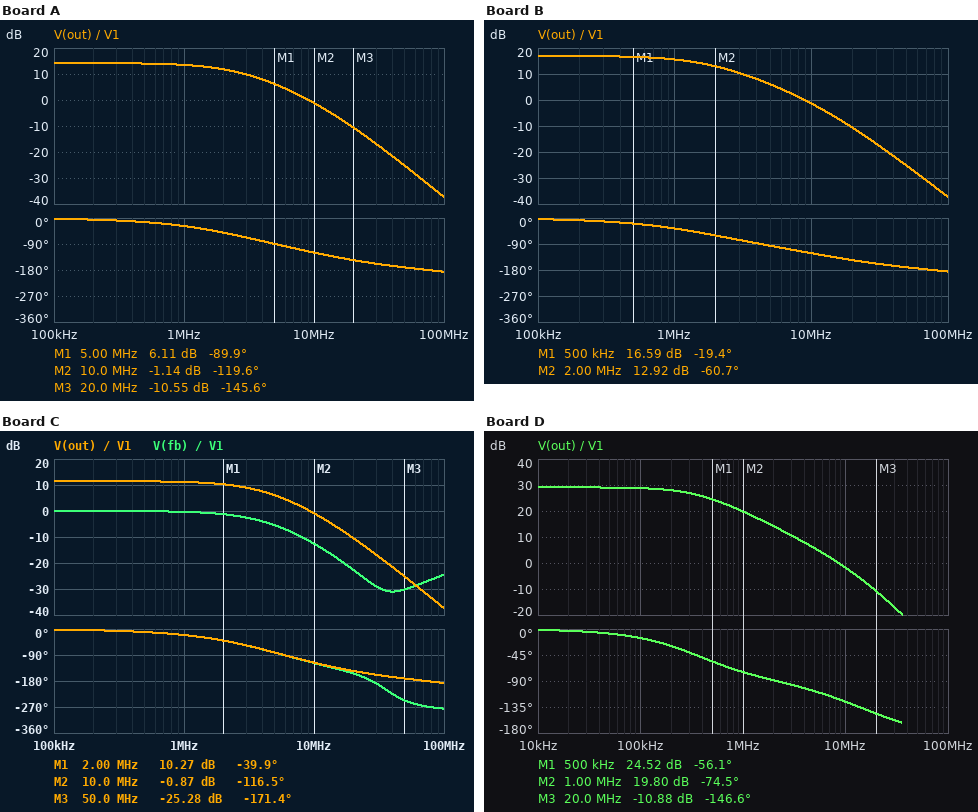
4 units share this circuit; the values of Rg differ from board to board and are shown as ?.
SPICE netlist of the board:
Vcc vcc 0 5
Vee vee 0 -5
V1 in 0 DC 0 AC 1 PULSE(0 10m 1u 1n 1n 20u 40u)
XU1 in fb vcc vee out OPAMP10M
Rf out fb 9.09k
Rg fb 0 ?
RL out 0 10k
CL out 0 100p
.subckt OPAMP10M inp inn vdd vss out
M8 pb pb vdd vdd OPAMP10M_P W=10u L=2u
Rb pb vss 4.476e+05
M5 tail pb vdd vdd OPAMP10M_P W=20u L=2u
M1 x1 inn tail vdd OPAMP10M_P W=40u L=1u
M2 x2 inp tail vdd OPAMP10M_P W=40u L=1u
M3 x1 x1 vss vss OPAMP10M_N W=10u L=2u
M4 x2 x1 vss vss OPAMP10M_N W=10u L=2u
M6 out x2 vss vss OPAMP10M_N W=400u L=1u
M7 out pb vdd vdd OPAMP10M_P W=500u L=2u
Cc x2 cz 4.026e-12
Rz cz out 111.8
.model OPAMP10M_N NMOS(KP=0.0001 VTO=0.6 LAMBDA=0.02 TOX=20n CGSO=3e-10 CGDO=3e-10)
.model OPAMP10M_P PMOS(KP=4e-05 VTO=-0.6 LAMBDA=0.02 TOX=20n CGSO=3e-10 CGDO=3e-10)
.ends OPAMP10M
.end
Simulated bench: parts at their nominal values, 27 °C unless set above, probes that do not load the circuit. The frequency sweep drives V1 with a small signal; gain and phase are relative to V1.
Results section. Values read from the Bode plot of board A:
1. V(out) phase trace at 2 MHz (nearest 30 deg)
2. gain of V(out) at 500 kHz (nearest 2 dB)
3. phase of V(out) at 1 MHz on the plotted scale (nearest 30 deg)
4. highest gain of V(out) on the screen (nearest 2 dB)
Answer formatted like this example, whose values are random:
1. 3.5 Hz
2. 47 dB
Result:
1. -60 deg
2. 14 dB
3. -30 deg
4. 14 dB
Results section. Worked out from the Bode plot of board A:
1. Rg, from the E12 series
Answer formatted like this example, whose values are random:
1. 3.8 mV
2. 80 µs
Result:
1. 2.2 kΩ
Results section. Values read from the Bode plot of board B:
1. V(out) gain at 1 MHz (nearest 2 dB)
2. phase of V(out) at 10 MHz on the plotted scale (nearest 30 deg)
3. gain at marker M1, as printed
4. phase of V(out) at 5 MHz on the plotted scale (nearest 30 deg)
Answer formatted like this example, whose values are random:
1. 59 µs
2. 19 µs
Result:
1. 16 dB
2. -120 deg
3. 16.59 dB
4. -90 deg
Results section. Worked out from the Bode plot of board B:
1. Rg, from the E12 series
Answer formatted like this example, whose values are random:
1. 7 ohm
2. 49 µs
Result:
1. 1.5 kΩ
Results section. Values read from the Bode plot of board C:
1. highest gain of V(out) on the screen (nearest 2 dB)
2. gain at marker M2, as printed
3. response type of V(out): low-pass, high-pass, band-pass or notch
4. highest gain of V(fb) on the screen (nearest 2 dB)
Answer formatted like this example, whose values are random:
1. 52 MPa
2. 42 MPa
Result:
1. 12 dB
2. -0.87 dB
3. low-pass
4. 0 dB
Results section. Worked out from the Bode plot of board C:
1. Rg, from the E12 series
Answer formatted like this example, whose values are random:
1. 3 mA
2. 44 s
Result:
1. 3.3 kΩ
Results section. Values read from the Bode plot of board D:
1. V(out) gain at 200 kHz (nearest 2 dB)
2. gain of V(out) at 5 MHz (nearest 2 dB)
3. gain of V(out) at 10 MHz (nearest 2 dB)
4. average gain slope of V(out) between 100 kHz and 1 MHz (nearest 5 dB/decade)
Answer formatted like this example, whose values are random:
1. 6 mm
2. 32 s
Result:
1. 28 dB
2. 6 dB
3. -2 dB
4. -10 dB/decade
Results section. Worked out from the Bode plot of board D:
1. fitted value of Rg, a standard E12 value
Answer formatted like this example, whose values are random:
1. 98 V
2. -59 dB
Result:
1. 330 Ω
